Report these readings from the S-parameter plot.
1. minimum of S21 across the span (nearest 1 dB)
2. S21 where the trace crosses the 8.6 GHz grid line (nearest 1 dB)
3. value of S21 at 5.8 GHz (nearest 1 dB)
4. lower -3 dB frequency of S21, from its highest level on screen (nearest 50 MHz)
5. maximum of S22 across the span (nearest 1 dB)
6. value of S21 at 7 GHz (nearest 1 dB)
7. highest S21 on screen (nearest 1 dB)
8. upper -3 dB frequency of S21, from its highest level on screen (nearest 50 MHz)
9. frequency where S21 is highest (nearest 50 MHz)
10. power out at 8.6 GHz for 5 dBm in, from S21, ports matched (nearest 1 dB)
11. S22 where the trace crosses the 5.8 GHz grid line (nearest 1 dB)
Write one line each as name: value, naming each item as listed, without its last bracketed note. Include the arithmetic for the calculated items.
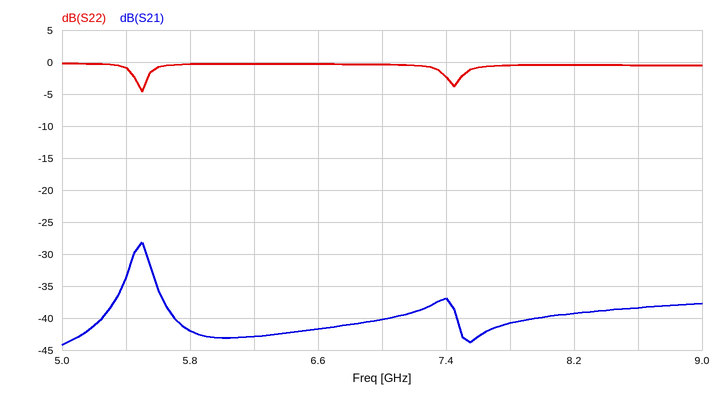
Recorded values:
minimum of S21 across the span: -44 dB
S21 where the trace crosses the 8.6 GHz grid line: -38 dB
value of S21 at 5.8 GHz: -42 dB
lower -3 dB frequency of S21, from its highest level on screen: 5.45 GHz
maximum of S22 across the span: 0 dB
value of S21 at 7 GHz: -40 dB
highest S21 on screen: -28 dB
upper -3 dB frequency of S21, from its highest level on screen: 5.55 GHz
frequency where S21 is highest: 5.50 GHz
power out at 8.6 GHz for 5 dBm in, from S21, ports matched: 5 dBm + (-38 dB) = -33 dBm
S22 where the trace crosses the 5.8 GHz grid line: 0 dB
